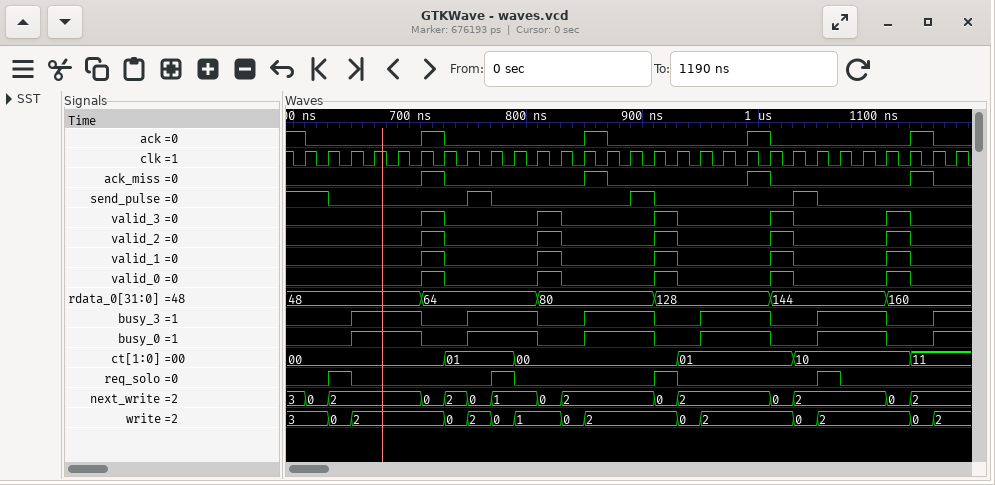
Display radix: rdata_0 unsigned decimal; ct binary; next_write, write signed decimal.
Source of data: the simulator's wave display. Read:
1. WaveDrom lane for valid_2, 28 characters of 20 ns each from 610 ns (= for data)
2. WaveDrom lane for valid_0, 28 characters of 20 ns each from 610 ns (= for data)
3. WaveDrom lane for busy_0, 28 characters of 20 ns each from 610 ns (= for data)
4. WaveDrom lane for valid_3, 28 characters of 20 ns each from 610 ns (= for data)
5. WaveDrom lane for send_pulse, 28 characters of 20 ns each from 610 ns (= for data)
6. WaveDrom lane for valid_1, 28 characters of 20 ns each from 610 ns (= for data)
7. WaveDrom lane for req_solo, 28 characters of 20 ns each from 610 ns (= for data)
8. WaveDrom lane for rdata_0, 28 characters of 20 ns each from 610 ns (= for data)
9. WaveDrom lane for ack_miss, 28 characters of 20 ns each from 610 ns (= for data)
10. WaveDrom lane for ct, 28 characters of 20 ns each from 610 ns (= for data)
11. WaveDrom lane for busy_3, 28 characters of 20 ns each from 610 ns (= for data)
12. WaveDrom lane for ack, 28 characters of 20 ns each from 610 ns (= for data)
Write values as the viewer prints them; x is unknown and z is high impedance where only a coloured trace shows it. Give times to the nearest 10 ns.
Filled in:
{name: 'valid_2', wave: '0....10...10...10...10...10.'}
{name: 'valid_0', wave: '0....10...10...10...10...10.'}
{name: 'busy_0', wave: '0.1..0.1..0.1..0.1..0.1..0.1'}
{name: 'valid_3', wave: '0....10...10...10...10...10.'}
{name: 'send_pulse', wave: '10.....10.....10.....10.....'}
{name: 'valid_1', wave: '0....10...10...10...10...10.'}
{name: 'req_solo', wave: '010.....10.....10.....10....'}
{name: 'rdata_0', wave: '=....=....=....=....=....=..', data: '48 64 80 128 144 160'}
{name: 'ack_miss', wave: '0....10.....10.....10.....10'}
{name: 'ct', wave: '=.....=..=......=....=....=.', data: '00 01 00 01 10 11'}
{name: 'busy_3', wave: '0.1..0.1..0.1..0.1..0.1..0.1'}
{name: 'ack', wave: '0....10.....10.....10.....10'}
